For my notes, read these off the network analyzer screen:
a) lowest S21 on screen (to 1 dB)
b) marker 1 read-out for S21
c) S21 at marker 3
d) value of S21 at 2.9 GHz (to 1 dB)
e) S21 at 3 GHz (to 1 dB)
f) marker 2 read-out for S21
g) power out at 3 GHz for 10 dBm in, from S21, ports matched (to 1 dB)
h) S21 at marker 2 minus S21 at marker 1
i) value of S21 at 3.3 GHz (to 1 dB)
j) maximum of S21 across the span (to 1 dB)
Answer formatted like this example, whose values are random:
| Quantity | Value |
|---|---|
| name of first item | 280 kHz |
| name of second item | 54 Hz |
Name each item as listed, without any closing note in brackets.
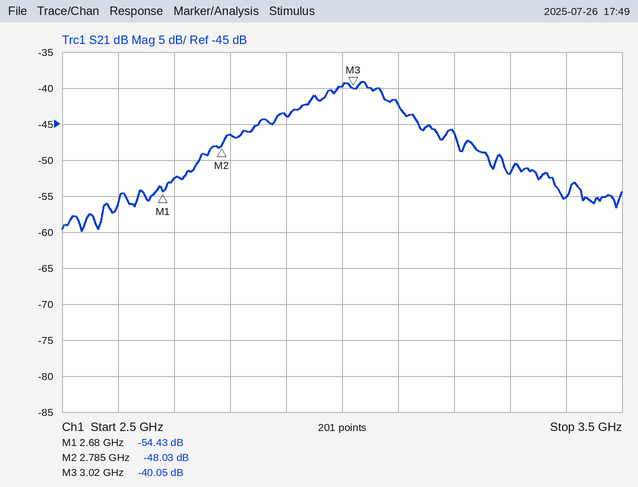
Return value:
| Quantity | Value |
|---|---|
| lowest S21 on screen | -60 dB |
| marker 1 read-out for S21 | -54.43 dB |
| S21 at marker 3 | -40.05 dB |
| value of S21 at 2.9 GHz | -44 dB |
| S21 at 3 GHz | -40 dB |
| marker 2 read-out for S21 | -48.03 dB |
| power out at 3 GHz for 10 dBm in, from S21, ports matched | -30 dBm |
| S21 at marker 2 minus S21 at marker 1 | 6.40 dB |
| value of S21 at 3.3 GHz | -52 dB |
| maximum of S21 across the span | -39 dB |
